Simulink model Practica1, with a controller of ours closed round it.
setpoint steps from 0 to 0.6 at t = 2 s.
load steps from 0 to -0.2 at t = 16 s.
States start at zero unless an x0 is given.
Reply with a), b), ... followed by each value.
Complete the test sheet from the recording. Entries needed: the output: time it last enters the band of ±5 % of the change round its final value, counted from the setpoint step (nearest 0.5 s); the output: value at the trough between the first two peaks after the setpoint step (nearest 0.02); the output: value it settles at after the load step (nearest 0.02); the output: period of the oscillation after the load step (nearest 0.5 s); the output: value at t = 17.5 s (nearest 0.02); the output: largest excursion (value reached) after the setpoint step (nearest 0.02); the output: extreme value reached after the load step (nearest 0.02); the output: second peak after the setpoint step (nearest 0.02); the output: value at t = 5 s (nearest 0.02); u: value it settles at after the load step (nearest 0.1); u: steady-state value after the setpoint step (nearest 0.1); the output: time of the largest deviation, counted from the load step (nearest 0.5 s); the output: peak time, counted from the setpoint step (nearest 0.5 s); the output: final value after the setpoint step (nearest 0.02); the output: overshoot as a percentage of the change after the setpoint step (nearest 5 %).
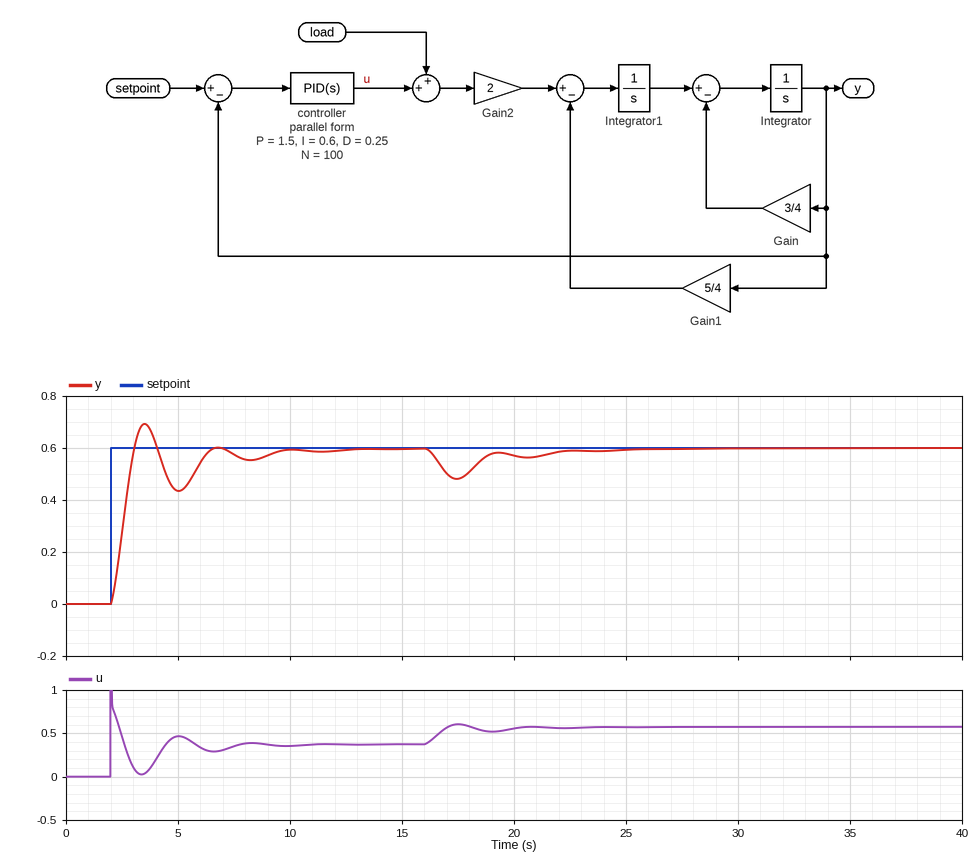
a) 7.0 s
b) 0.44
c) 0.60
d) 3.0 s
e) 0.48
f) 0.70
g) 0.48
h) 0.60
i) 0.44
j) 0.6
k) 0.4
l) 1.5 s
m) 1.5 s
n) 0.60
o) 15 %
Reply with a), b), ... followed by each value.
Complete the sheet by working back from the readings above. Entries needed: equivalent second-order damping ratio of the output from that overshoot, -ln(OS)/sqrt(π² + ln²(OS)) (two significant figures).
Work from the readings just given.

a) 0.52
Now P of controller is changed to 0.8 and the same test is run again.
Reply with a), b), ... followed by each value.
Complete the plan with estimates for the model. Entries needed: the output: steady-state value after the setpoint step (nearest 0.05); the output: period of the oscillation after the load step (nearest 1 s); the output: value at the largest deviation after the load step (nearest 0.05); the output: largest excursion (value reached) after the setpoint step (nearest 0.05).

a) 0.60
b) 4 s
c) 0.45
d) 0.65
